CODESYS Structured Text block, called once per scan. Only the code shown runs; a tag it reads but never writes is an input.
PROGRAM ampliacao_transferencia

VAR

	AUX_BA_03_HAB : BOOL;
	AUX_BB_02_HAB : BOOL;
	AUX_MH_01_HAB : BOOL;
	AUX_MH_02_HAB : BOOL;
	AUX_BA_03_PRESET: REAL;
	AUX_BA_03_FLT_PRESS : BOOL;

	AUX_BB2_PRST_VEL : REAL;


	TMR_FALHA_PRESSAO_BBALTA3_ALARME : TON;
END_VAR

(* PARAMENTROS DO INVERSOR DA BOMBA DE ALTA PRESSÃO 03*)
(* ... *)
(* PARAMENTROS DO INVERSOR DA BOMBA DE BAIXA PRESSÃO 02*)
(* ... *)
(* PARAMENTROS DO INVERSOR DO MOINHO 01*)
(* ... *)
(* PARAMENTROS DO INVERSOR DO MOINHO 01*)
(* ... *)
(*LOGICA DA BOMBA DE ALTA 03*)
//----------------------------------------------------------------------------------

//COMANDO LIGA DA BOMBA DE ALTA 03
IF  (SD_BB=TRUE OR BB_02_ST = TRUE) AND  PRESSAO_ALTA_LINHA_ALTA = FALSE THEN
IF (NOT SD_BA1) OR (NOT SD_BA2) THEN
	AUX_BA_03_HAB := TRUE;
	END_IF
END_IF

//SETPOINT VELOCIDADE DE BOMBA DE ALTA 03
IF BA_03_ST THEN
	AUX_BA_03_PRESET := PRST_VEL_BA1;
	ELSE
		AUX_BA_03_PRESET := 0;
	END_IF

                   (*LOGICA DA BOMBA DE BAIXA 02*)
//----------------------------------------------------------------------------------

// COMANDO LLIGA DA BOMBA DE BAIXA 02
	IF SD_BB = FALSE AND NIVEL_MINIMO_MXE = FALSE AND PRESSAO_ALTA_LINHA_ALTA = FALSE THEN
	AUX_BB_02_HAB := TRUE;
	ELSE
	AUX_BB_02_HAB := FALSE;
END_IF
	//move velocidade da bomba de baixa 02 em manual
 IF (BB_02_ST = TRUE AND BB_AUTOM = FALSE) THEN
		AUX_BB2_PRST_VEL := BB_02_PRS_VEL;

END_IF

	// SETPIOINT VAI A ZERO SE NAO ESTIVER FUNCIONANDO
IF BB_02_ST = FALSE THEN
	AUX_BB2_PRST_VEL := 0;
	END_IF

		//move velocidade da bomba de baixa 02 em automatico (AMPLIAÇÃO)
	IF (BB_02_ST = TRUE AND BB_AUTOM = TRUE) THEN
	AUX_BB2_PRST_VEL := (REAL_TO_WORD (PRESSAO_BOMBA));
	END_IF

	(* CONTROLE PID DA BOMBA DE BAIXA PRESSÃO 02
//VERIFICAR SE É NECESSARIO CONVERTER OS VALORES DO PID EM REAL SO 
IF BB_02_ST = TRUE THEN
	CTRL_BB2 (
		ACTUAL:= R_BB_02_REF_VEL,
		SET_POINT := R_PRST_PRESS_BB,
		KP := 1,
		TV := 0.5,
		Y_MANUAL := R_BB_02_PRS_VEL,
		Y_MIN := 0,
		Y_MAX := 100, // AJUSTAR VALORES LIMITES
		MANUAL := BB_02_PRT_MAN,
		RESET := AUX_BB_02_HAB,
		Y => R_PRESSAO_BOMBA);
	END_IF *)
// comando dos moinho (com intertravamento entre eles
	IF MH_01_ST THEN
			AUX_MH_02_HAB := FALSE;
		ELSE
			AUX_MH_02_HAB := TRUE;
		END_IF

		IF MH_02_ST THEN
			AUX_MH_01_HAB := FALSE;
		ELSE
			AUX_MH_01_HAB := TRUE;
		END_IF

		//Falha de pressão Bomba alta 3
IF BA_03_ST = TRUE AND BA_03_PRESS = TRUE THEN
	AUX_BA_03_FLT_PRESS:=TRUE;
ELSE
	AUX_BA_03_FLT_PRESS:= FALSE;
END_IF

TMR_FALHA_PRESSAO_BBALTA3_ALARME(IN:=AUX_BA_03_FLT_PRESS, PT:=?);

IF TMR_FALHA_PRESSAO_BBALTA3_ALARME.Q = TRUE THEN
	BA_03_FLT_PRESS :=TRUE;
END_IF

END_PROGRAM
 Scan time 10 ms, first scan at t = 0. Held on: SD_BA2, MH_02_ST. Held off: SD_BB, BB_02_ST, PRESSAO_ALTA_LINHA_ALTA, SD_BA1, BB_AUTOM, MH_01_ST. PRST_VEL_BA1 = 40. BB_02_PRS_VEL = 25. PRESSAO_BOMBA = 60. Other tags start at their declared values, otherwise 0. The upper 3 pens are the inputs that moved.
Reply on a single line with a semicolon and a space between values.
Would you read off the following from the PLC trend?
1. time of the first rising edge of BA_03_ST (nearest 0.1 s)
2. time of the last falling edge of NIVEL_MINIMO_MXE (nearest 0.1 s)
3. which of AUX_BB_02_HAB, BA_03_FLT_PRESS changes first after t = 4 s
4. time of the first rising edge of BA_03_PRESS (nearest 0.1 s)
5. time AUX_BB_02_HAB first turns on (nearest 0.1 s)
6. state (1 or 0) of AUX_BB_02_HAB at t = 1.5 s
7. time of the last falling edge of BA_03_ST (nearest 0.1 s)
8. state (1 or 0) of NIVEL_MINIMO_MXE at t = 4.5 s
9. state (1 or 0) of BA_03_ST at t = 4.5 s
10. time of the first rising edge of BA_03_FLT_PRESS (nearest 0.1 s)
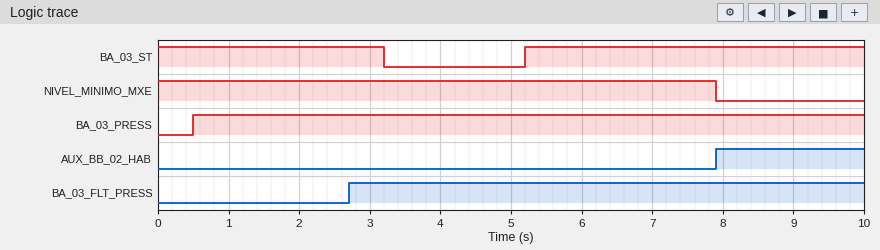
5.2 s; 7.9 s; AUX_BB_02_HAB; 0.5 s; 7.9 s; 0; 3.2 s; 1; 0; 2.7 s
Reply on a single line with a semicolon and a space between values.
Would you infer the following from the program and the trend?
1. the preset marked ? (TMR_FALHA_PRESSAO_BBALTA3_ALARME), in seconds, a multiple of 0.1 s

2.2 s
